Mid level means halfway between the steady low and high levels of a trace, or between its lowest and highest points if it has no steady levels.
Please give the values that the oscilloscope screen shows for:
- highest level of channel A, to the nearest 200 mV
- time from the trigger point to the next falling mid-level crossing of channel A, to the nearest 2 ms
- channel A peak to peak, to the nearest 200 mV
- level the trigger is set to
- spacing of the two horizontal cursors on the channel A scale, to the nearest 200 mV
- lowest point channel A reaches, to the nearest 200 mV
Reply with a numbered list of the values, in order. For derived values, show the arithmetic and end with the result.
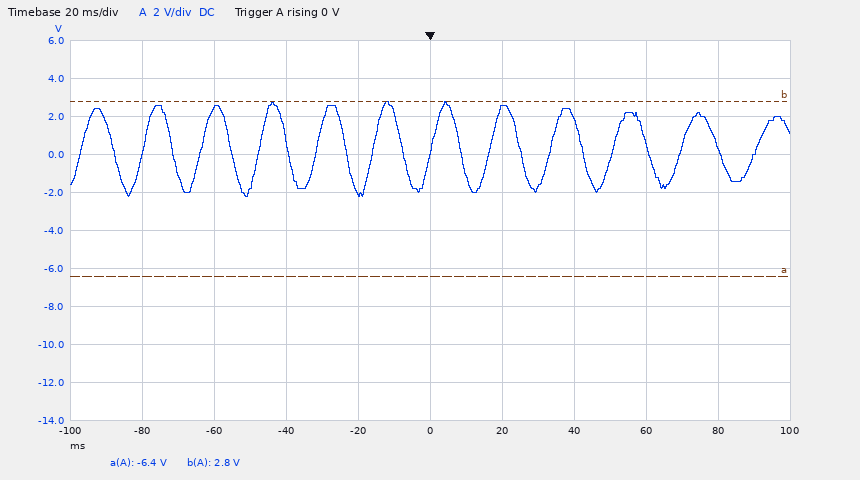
1. 2.8 V
2. 8 ms
3. 2.8 V − (-2.2 V) = 5.0 V
4. 0 V
5. 9.2 V
6. -2.2 V
